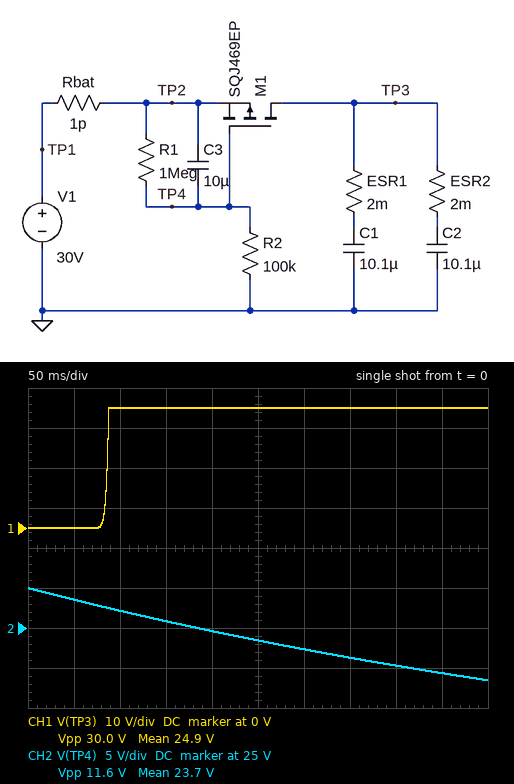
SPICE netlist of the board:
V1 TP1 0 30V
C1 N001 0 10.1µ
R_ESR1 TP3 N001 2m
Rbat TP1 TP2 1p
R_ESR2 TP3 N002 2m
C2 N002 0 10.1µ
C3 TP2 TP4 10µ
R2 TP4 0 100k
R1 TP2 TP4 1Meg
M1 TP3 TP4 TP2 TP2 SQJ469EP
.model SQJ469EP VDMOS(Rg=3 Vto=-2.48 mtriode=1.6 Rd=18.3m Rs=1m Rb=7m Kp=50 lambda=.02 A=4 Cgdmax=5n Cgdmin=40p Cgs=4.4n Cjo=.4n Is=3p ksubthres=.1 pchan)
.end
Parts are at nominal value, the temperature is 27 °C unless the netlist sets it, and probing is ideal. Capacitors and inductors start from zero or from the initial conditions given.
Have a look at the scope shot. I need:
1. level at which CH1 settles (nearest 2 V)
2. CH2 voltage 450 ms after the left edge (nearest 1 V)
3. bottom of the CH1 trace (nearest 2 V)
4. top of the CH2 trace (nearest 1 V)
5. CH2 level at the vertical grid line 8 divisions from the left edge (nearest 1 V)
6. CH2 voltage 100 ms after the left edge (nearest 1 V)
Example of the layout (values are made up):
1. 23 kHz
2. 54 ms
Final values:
1. 30 V
2. 19 V
3. 0 V
4. 30 V
5. 20 V
6. 27 V
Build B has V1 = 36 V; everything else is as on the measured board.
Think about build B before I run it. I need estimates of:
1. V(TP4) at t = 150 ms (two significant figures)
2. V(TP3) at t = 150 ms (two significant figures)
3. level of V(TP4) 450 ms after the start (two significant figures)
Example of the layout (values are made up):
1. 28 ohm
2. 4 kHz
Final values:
1. 31 V
2. 36 V
3. 23 V
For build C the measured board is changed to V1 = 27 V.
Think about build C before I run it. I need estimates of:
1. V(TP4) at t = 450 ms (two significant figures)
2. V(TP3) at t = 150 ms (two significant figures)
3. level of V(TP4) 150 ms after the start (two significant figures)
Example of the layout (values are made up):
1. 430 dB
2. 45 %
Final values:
1. 17 V
2. 27 V
3. 23 V
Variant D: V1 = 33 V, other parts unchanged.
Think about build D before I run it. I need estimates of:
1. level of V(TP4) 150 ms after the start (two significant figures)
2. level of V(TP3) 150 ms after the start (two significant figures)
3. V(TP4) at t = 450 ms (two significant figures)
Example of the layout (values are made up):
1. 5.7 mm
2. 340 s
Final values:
1. 28 V
2. 33 V
3. 21 V
